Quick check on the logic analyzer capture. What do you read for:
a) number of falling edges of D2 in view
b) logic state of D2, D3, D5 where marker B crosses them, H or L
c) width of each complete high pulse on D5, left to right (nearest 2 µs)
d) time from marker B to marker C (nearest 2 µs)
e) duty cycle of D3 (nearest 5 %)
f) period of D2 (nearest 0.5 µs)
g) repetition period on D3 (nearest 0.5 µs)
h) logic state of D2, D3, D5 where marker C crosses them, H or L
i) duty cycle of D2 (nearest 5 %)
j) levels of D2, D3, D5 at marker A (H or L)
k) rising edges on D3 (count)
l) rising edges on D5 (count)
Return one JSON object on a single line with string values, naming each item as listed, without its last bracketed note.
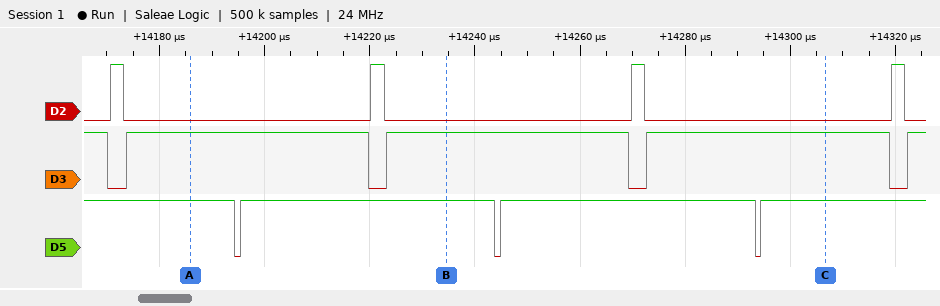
{"number of falling edges of D2 in view": "4", "logic state of D2, D3, D5 where marker B crosses them, H or L": "D2=L, D3=H, D5=H", "width of each complete high pulse on D5, left to right": "48 µs, 48 µs", "time from marker B to marker C": "72 µs", "duty cycle of D3": "95 %", "period of D2": "49.5 µs", "repetition period on D3": "49.5 µs", "logic state of D2, D3, D5 where marker C crosses them, H or L": "D2=L, D3=H, D5=H", "duty cycle of D2": "5 %", "levels of D2, D3, D5 at marker A": "D2=L, D3=H, D5=H", "rising edges on D3": "4", "rising edges on D5": "3"}
